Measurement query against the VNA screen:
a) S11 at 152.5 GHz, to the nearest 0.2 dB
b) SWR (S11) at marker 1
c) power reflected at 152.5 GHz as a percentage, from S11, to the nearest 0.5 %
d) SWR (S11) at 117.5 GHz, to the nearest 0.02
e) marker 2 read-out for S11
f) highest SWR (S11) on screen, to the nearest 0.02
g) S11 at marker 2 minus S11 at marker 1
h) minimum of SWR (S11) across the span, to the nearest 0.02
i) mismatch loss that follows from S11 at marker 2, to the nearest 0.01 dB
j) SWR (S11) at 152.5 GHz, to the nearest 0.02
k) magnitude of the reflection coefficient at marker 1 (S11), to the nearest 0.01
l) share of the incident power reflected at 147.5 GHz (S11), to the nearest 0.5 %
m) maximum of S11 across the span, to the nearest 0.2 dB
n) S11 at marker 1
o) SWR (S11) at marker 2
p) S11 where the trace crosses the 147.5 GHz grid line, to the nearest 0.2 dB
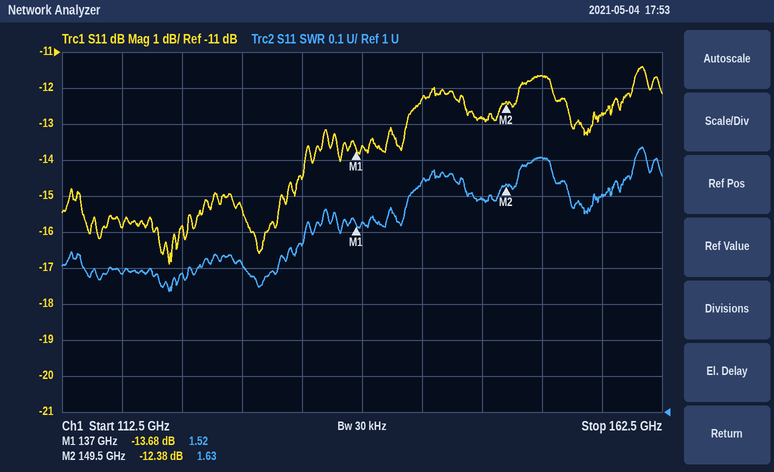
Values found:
-11.6 dB
1.52
7.0 %
1.38
-12.38 dB
1.74
1.30 dB
1.34
0.26 dB
1.70
0.21
5.0 %
-11.4 dB
-13.68 dB
1.63
-12.8 dB
